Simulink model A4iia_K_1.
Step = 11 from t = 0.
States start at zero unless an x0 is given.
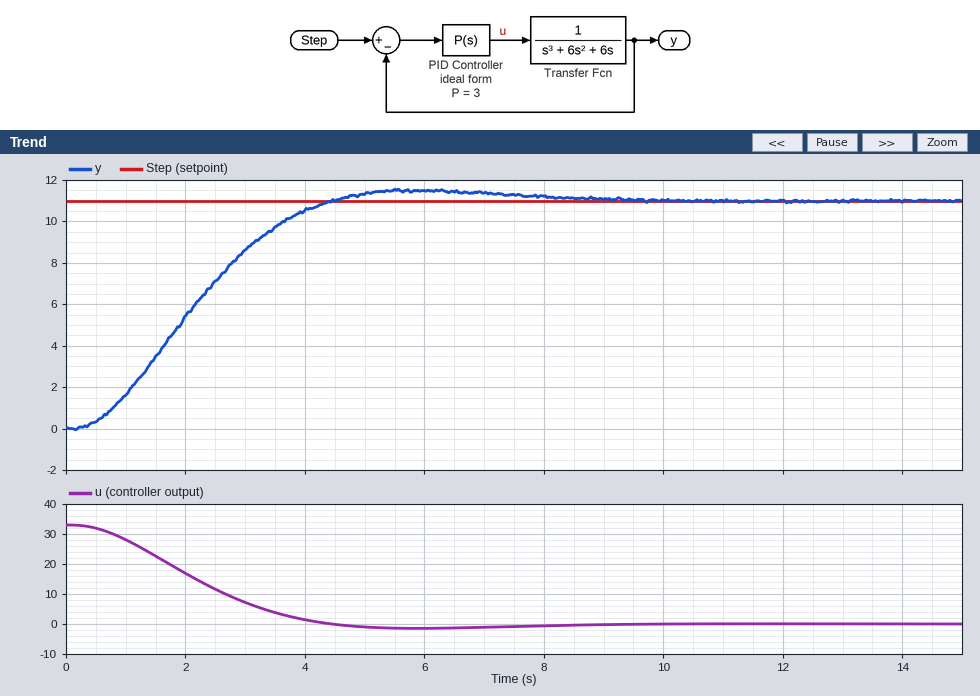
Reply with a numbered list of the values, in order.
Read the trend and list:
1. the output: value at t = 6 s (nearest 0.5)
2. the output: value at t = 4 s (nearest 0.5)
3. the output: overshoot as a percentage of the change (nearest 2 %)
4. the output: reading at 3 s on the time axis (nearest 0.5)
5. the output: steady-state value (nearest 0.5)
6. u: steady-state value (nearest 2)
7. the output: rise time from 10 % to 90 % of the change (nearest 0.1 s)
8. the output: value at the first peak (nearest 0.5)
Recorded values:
1. 11.5
2. 10.5
3. 4 %
4. 8.5
5. 11.0
6. 0
7. 2.8 s
8. 11.5
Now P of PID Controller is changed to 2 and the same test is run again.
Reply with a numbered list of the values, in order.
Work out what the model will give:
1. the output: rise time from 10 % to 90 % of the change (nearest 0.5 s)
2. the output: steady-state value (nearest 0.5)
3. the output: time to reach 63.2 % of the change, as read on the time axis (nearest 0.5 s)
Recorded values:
1. 4.5 s
2. 11.0
3. 3.5 s
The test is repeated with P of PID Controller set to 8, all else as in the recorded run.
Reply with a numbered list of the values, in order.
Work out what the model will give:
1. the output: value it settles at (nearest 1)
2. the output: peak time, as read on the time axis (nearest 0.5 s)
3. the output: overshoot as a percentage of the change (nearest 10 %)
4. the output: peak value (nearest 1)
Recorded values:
1. 11
2. 3.0 s
3. 30 %
4. 14
